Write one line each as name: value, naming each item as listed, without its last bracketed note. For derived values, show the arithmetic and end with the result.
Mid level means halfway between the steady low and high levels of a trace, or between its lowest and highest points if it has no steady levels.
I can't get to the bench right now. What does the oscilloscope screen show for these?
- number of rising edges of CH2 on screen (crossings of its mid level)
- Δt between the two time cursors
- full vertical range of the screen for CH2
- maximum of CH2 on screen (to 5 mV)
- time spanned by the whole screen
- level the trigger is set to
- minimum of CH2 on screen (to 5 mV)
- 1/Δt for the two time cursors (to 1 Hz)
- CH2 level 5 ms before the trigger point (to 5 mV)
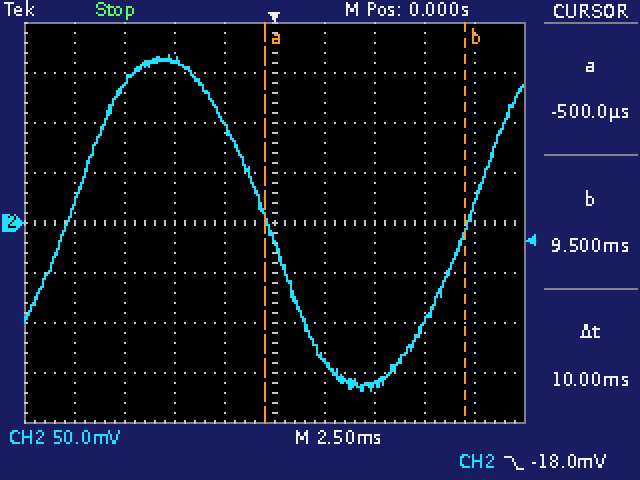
number of rising edges of CH2 on screen: 2
Δt between the two time cursors: 10 ms
full vertical range of the screen for CH2: 400 mV
maximum of CH2 on screen: 170 mV
time spanned by the whole screen: 25 ms
level the trigger is set to: -18.0 mV
minimum of CH2 on screen: -170 mV
1/Δt for the two time cursors: 1 / 10 ms ≈ 100 Hz
CH2 level 5 ms before the trigger point: 165 mV
